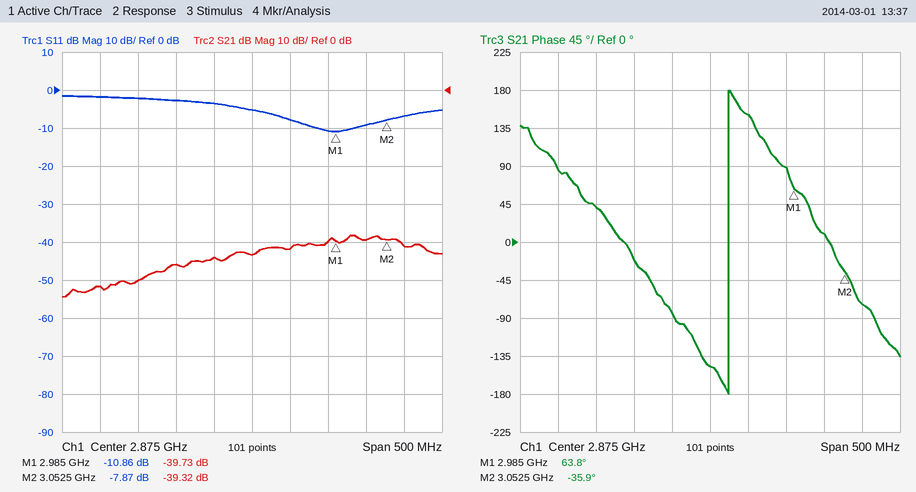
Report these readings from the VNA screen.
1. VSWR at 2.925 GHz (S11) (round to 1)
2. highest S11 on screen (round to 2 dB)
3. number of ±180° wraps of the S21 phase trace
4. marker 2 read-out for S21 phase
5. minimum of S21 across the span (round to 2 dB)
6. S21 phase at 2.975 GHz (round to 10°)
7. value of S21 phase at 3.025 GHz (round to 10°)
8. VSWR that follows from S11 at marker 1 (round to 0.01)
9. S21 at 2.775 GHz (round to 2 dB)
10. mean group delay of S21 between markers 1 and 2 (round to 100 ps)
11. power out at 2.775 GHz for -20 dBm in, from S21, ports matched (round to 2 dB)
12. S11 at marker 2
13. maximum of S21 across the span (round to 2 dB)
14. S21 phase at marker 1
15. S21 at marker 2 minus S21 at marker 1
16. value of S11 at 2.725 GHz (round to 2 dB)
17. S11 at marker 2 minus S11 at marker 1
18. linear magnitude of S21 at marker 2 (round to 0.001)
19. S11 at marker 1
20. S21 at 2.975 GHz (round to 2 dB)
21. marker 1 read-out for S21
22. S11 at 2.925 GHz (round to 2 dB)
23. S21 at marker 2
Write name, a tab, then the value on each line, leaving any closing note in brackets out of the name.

VSWR at 2.925 GHz (S11)	2
highest S11 on screen	-2 dB
number of ±180° wraps of the S21 phase trace	1
marker 2 read-out for S21 phase	-35.9°
minimum of S21 across the span	-54 dB
S21 phase at 2.975 GHz	90°
value of S21 phase at 3.025 GHz	10°
VSWR that follows from S11 at marker 1	1.80
S21 at 2.775 GHz	-46 dB
mean group delay of S21 between markers 1 and 2	4.1 ns
power out at 2.775 GHz for -20 dBm in, from S21, ports matched	-66 dBm
S11 at marker 2	-7.87 dB
maximum of S21 across the span	-38 dB
S21 phase at marker 1	63.8°
S21 at marker 2 minus S21 at marker 1	0.41 dB
value of S11 at 2.725 GHz	-2 dB
S11 at marker 2 minus S11 at marker 1	2.99 dB
linear magnitude of S21 at marker 2	0.011
S11 at marker 1	-10.86 dB
S21 at 2.975 GHz	-40 dB
marker 1 read-out for S21	-39.73 dB
S11 at 2.925 GHz	-8 dB
S21 at marker 2	-39.32 dB
